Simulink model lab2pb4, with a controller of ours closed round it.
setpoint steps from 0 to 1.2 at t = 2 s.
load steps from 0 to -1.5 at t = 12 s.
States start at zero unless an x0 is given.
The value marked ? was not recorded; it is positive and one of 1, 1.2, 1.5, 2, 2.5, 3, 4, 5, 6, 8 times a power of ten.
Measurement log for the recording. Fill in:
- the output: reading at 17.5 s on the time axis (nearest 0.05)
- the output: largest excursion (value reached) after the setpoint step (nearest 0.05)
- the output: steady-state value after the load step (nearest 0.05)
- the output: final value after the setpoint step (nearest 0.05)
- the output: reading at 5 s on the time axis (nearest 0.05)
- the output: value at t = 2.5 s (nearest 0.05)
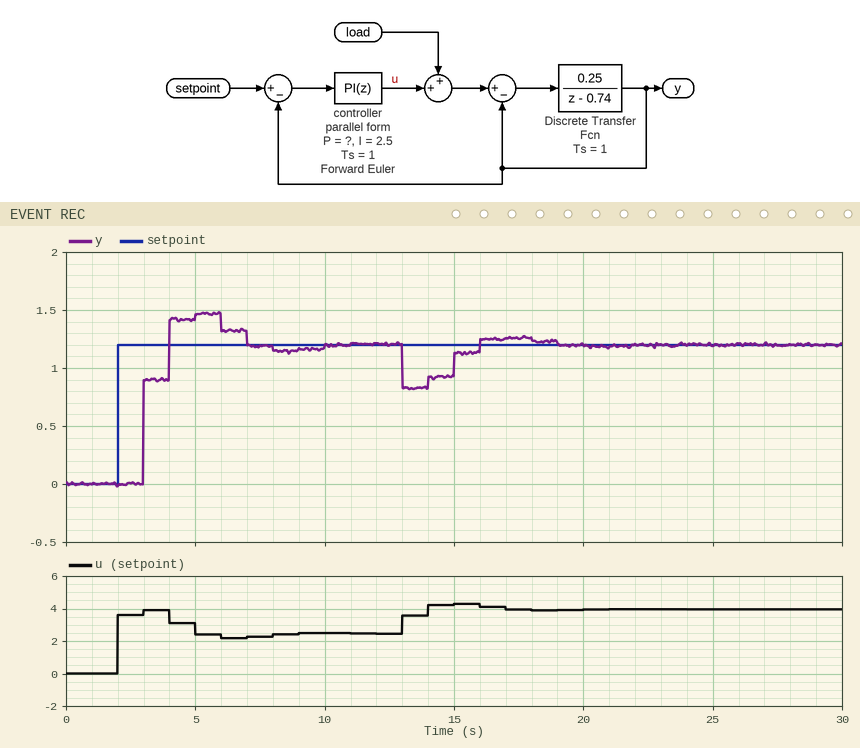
1.25
1.45
1.20
1.20
1.45
0.00
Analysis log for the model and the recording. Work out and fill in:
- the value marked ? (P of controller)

3
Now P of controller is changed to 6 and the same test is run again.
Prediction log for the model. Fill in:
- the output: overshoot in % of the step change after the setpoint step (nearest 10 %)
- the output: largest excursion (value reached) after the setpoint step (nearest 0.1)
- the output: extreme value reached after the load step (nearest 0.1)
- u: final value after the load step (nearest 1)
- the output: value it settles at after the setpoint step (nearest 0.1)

50 %
1.8
0.8
4
1.2
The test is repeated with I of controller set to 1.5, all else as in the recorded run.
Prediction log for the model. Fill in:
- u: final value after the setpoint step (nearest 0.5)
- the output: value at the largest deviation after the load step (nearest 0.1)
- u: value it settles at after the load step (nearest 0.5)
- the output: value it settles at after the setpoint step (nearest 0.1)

2.5
0.8
4.0
1.2
